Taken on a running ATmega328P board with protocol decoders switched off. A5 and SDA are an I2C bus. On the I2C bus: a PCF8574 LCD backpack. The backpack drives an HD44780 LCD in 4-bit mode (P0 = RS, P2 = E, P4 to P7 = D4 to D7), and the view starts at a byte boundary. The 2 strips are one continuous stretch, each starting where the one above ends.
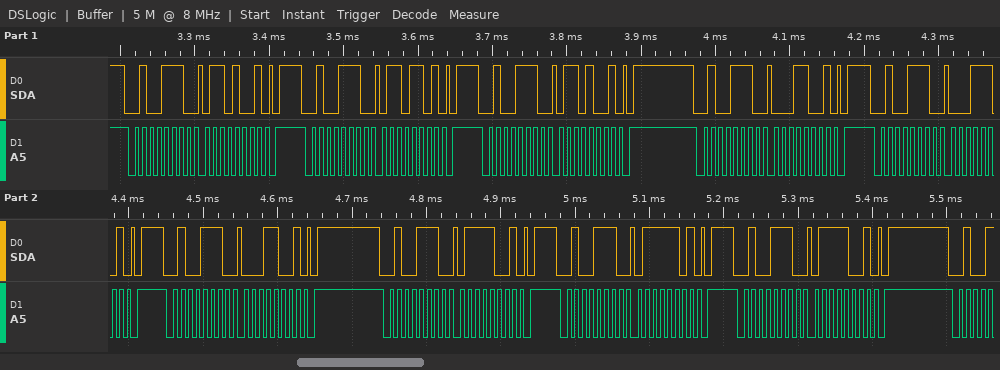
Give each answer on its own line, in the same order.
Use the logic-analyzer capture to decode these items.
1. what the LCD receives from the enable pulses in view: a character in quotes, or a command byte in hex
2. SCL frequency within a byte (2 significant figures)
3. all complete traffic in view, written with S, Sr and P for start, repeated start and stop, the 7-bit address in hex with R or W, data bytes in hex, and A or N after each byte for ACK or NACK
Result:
'a'
100 kHz
S 27W A 69 A P S 27W A 6D A P S 27W A 69 A P S 27W A 19 A P S 27W A 1D A P S 27W A 19 A P S 27W A 79 A P S 27W A 7D A P S 27W A 79 A P
